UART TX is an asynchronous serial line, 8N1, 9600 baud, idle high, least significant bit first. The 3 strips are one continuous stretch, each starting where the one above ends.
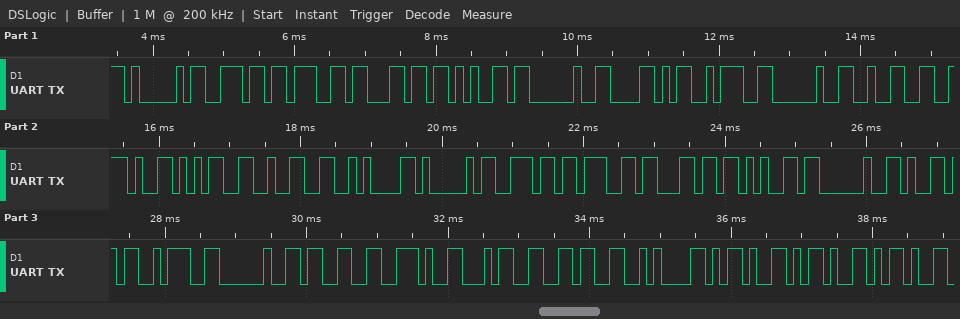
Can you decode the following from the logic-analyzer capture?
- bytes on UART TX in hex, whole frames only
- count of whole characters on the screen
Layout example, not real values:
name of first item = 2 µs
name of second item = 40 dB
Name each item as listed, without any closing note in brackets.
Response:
bytes on UART TX in hex, whole frames only = 41 6E 67 6C 65 20 58 3A 20 32 2E 35 32 0A 41 6E 67 6C 65 20 59 3A 20 33 2E 34 36 0A 2D 2D 2D
count of whole characters on the screen = 31
